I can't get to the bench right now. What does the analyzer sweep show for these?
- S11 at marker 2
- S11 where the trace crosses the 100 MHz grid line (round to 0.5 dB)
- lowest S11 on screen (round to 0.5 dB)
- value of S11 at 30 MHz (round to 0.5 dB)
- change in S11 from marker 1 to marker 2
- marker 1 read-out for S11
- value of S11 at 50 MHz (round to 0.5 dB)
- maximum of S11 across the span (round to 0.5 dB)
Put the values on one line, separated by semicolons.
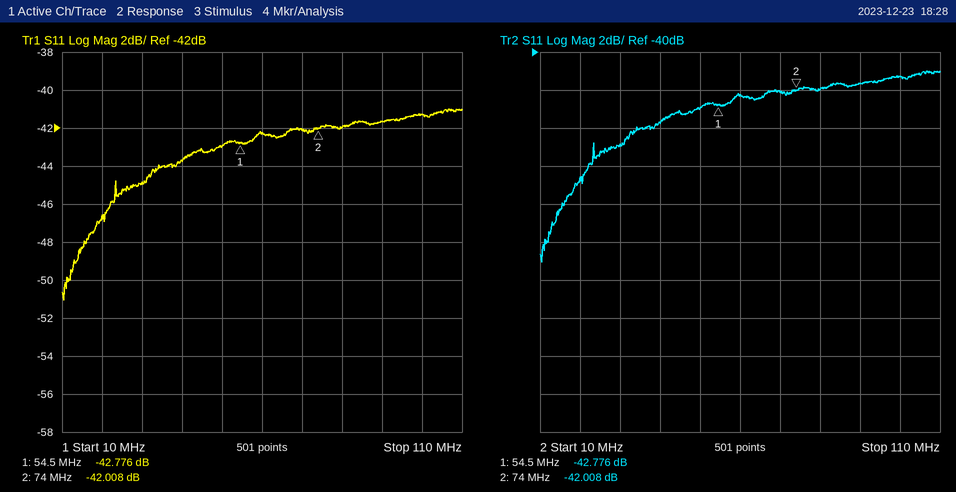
-42.008 dB; -41.5 dB; -51.0 dB; -45.0 dB; 0.768 dB; -42.776 dB; -43.0 dB; -41.0 dB
